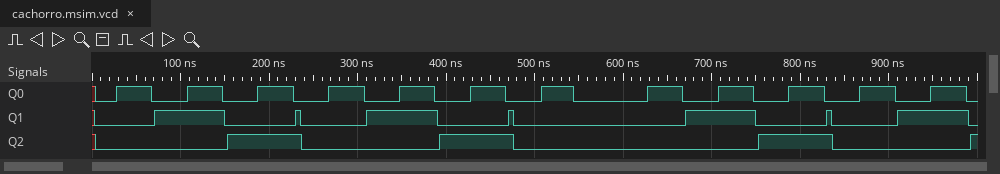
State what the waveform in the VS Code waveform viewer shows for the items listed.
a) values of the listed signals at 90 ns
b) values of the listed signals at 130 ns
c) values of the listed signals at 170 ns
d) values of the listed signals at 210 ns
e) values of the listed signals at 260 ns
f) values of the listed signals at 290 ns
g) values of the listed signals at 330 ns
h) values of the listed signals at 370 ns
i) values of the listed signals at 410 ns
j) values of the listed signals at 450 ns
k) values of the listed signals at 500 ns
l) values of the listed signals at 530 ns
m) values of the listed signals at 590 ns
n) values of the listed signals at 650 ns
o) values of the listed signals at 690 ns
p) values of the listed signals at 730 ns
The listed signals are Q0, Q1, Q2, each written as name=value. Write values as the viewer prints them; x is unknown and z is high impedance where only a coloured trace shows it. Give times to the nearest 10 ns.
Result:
Q0=0, Q1=1, Q2=0
Q0=1, Q1=1, Q2=0
Q0=0, Q1=0, Q2=1
Q0=1, Q1=0, Q2=1
Q0=0, Q1=0, Q2=0
Q0=1, Q1=0, Q2=0
Q0=0, Q1=1, Q2=0
Q0=1, Q1=1, Q2=0
Q0=0, Q1=0, Q2=1
Q0=1, Q1=0, Q2=1
Q0=0, Q1=0, Q2=0
Q0=1, Q1=0, Q2=0
Q0=0, Q1=0, Q2=0
Q0=1, Q1=0, Q2=0
Q0=0, Q1=1, Q2=0
Q0=1, Q1=1, Q2=0
